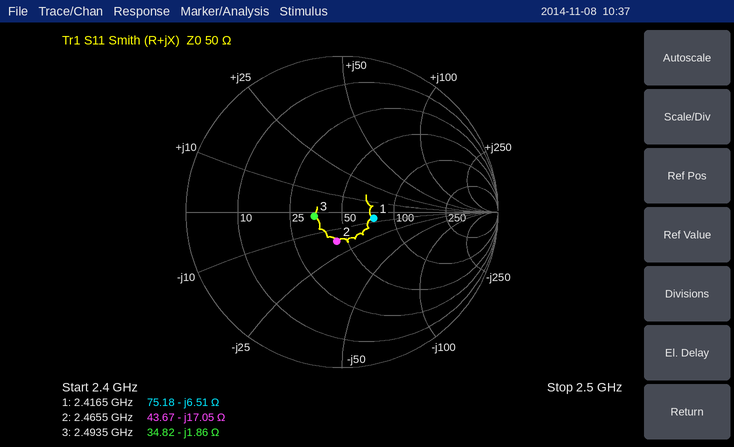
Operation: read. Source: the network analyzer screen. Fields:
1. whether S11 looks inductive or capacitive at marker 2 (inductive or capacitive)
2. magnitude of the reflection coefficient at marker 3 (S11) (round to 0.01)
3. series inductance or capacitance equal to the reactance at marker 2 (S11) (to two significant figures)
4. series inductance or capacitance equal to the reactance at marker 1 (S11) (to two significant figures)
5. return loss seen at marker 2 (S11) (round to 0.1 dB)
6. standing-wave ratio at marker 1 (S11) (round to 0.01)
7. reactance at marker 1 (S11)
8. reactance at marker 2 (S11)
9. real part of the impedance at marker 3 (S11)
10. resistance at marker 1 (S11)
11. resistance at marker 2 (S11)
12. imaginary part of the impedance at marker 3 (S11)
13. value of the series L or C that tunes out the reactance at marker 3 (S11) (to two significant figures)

capacitive
0.18
3.8 pF
10 pF
14.4 dB
1.52
-6.51 Ω
-17.05 Ω
34.82 Ω
75.18 Ω
43.67 Ω
-1.86 Ω
120 pH
